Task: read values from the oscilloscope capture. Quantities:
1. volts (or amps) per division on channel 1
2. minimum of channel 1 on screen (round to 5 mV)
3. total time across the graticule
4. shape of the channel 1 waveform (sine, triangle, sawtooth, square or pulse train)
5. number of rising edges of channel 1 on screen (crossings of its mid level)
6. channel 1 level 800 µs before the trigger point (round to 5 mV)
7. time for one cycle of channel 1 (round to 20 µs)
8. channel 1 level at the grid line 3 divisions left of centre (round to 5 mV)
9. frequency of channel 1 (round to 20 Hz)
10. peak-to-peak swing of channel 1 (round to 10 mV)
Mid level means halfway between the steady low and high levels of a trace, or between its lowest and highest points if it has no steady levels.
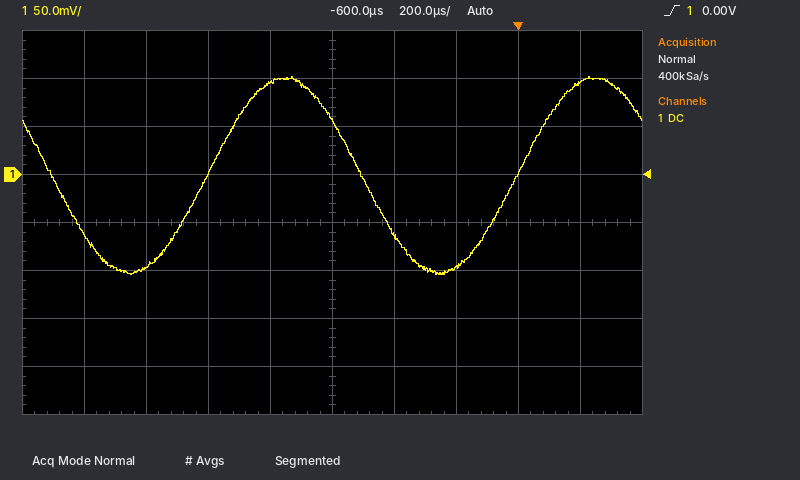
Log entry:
50 mV
-105 mV
2 ms
sine
2
95 mV
1.00 ms
-95 mV
1.00 kHz
210 mV
